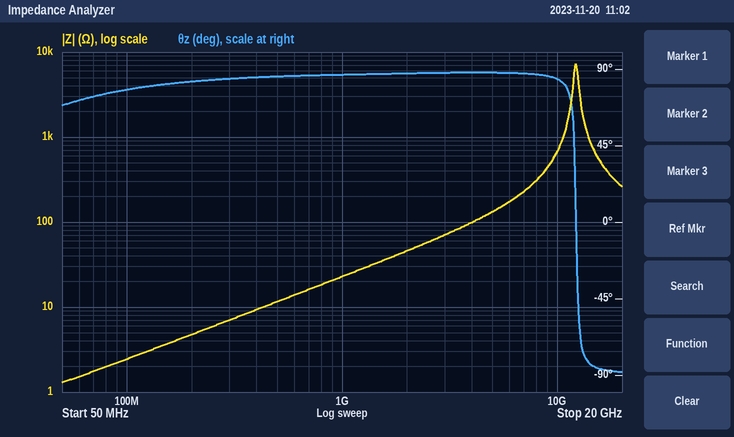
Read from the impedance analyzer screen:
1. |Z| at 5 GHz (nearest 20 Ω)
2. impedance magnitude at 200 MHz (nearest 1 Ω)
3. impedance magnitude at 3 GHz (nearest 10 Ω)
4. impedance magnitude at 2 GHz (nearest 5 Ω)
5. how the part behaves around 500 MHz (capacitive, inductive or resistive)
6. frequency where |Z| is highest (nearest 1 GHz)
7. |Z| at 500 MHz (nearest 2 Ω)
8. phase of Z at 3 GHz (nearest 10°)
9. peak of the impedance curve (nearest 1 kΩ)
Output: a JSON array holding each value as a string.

["140 Ω", "5 Ω", "70 Ω", "45 Ω", "inductive", "12 GHz", "12 Ω", "90°", "7 kΩ"]
